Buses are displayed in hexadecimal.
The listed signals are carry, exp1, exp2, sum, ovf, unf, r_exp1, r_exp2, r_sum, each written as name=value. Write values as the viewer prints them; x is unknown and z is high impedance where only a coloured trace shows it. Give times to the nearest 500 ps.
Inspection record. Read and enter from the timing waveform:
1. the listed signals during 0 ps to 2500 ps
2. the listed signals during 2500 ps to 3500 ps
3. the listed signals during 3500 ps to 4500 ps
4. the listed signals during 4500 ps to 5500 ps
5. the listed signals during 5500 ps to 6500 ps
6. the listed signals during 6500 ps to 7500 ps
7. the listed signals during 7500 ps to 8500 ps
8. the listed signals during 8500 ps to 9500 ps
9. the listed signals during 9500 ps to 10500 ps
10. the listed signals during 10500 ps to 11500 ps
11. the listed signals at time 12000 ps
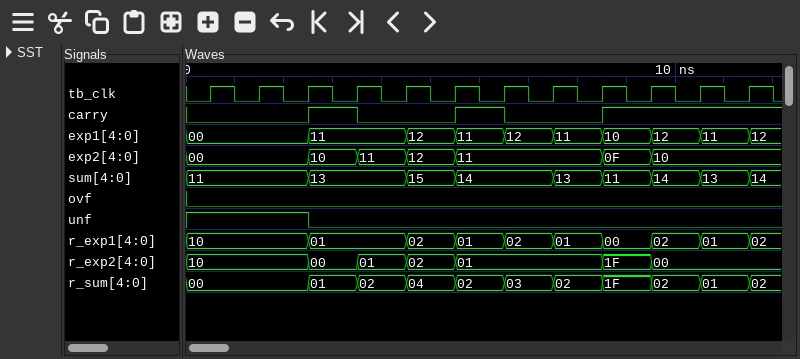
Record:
carry=0, exp1=00, exp2=00, sum=11, ovf=0, unf=1, r_exp1=10, r_exp2=10, r_sum=00
carry=1, exp1=11, exp2=10, sum=13, ovf=0, unf=0, r_exp1=01, r_exp2=00, r_sum=01
carry=0, exp1=11, exp2=11, sum=13, ovf=0, unf=0, r_exp1=01, r_exp2=01, r_sum=02
carry=0, exp1=12, exp2=12, sum=15, ovf=0, unf=0, r_exp1=02, r_exp2=02, r_sum=04
carry=1, exp1=11, exp2=11, sum=14, ovf=0, unf=0, r_exp1=01, r_exp2=01, r_sum=02
carry=0, exp1=12, exp2=11, sum=14, ovf=0, unf=0, r_exp1=02, r_exp2=01, r_sum=03
carry=0, exp1=11, exp2=11, sum=13, ovf=0, unf=0, r_exp1=01, r_exp2=01, r_sum=02
carry=1, exp1=10, exp2=0F, sum=11, ovf=0, unf=0, r_exp1=00, r_exp2=1F, r_sum=1F
carry=1, exp1=12, exp2=10, sum=14, ovf=0, unf=0, r_exp1=02, r_exp2=00, r_sum=02
carry=1, exp1=11, exp2=10, sum=13, ovf=0, unf=0, r_exp1=01, r_exp2=00, r_sum=01
carry=1, exp1=12, exp2=10, sum=14, ovf=0, unf=0, r_exp1=02, r_exp2=00, r_sum=02
